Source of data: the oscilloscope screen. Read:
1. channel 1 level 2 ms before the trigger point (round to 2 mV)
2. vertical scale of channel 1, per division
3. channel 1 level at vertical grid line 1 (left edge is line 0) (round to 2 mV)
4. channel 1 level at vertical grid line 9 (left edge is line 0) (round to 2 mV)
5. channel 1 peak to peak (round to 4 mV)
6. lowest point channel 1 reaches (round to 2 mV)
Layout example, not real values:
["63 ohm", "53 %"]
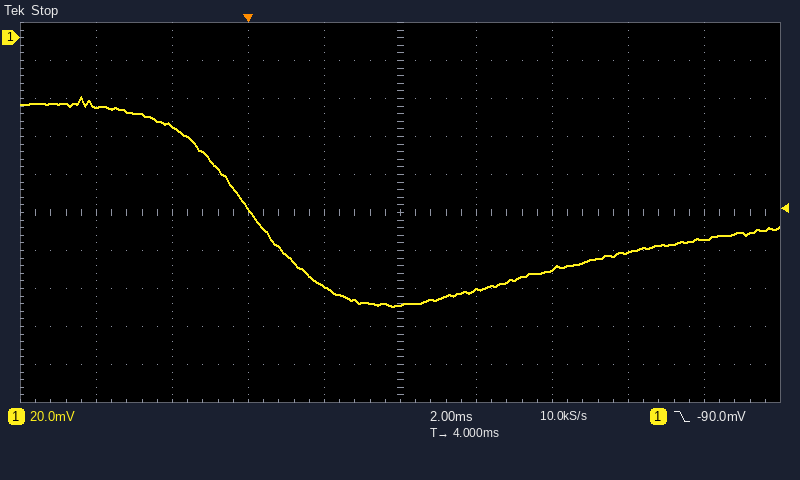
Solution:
["-46 mV", "20 mV", "-36 mV", "-106 mV", "112 mV", "-142 mV"]
